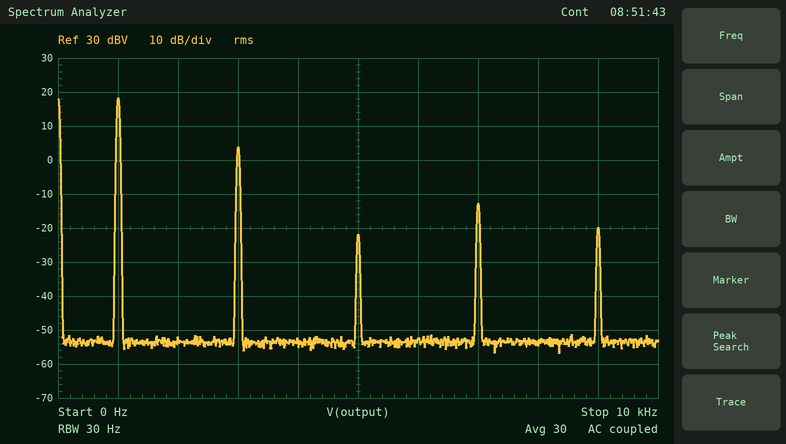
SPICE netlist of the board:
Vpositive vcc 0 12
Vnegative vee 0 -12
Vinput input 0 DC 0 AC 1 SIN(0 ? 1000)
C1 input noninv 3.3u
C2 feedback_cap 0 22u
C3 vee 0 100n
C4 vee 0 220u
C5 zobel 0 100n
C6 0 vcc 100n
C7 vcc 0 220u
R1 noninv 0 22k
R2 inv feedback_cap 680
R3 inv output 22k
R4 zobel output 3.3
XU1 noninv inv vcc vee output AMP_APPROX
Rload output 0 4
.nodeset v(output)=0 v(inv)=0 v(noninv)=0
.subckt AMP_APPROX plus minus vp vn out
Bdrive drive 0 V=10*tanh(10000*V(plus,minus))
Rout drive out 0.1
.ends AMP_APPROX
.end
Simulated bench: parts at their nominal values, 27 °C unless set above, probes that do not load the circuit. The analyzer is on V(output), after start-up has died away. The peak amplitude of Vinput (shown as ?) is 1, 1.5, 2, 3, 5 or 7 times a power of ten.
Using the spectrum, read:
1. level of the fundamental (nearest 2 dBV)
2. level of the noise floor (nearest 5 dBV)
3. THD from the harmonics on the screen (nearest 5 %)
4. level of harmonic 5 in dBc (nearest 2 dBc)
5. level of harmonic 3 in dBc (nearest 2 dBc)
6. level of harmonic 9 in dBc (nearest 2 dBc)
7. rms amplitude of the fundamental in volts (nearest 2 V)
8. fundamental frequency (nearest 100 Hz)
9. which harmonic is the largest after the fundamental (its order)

18 dBV
-55 dBV
20 %
-40 dBc
-14 dBc
-38 dBc
8 V
1.0 kHz
3
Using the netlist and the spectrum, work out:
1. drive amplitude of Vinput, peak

500 mV
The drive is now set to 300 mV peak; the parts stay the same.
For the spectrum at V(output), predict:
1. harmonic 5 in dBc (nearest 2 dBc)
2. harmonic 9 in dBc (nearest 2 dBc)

-48 dBc
-50 dBc
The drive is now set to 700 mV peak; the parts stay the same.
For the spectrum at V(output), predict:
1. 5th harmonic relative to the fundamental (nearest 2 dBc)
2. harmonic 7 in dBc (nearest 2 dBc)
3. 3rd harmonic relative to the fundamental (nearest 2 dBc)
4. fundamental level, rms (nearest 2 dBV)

-22 dBc
-42 dBc
-12 dBc
18 dBV
